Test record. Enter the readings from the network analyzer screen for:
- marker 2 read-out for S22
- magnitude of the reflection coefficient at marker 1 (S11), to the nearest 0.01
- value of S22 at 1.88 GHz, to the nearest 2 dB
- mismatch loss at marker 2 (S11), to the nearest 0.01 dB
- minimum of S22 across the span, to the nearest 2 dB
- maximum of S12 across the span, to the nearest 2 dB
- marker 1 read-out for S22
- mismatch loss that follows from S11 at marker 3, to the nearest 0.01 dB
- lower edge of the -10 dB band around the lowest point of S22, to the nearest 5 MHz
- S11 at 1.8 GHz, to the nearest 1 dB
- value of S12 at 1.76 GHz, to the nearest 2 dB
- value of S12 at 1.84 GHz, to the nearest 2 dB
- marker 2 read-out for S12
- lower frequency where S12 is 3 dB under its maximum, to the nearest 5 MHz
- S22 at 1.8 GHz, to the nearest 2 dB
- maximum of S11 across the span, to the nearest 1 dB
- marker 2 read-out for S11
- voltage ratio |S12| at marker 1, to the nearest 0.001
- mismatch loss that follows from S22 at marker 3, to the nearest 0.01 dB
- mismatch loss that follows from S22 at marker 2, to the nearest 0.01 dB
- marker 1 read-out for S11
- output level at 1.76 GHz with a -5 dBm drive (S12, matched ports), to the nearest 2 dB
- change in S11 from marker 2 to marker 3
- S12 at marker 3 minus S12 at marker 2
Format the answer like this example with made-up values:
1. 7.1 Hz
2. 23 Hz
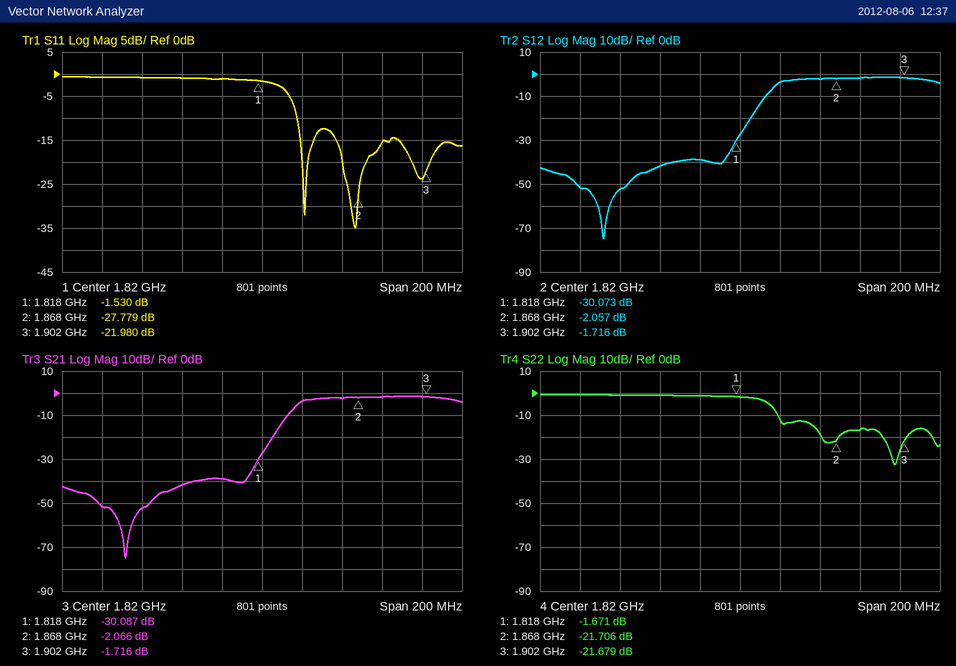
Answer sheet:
1. -21.706 dB
2. 0.84
3. -16 dB
4. 0.01 dB
5. -32 dB
6. -2 dB
7. -1.671 dB
8. 0.03 dB
9. 1.840 GHz
10. -1 dB
11. -52 dB
12. -4 dB
13. -2.057 dB
14. 1.840 GHz
15. -2 dB
16. -1 dB
17. -27.779 dB
18. 0.031
19. 0.03 dB
20. 0.03 dB
21. -1.530 dB
22. -58 dBm
23. 5.799 dB
24. 0.341 dB
